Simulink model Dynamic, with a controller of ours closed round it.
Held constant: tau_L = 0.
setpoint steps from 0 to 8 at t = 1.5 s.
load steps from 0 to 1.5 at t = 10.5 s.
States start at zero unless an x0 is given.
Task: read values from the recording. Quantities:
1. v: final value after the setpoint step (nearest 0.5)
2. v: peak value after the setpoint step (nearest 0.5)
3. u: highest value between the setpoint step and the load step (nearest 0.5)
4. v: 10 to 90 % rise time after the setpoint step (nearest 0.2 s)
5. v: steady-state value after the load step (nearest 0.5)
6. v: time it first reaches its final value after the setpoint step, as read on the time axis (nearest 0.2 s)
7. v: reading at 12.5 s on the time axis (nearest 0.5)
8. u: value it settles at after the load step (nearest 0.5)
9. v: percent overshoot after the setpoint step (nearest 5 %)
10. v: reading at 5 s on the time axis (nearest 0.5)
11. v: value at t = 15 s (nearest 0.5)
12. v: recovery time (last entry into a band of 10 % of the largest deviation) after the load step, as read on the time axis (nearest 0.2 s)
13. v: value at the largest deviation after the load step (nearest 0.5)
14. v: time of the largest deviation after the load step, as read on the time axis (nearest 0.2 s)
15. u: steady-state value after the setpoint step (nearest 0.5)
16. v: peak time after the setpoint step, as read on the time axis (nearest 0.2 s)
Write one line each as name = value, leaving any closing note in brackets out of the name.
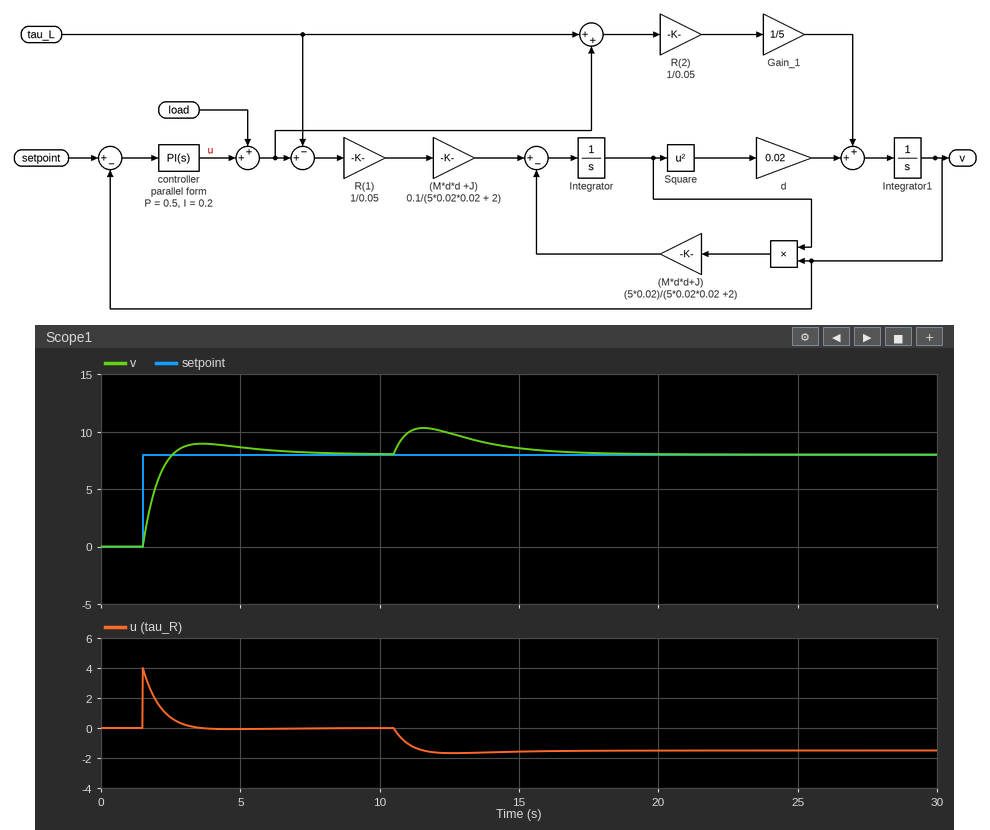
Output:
v: final value after the setpoint step = 8.0
v: peak value after the setpoint step = 9.0
u: highest value between the setpoint step and the load step = 4.0
v: 10 to 90 % rise time after the setpoint step = 0.8 s
v: steady-state value after the load step = 8.0
v: time it first reaches its final value after the setpoint step, as read on the time axis = 2.6 s
v: reading at 12.5 s on the time axis = 10.0
u: value it settles at after the load step = -1.5
v: percent overshoot after the setpoint step = 10 %
v: reading at 5 s on the time axis = 8.5
v: value at t = 15 s = 8.5
v: recovery time (last entry into a band of 10 % of the largest deviation) after the load step, as read on the time axis = 16.6 s
v: value at the largest deviation after the load step = 10.5
v: time of the largest deviation after the load step, as read on the time axis = 11.6 s
u: steady-state value after the setpoint step = 0.0
v: peak time after the setpoint step, as read on the time axis = 3.6 s
